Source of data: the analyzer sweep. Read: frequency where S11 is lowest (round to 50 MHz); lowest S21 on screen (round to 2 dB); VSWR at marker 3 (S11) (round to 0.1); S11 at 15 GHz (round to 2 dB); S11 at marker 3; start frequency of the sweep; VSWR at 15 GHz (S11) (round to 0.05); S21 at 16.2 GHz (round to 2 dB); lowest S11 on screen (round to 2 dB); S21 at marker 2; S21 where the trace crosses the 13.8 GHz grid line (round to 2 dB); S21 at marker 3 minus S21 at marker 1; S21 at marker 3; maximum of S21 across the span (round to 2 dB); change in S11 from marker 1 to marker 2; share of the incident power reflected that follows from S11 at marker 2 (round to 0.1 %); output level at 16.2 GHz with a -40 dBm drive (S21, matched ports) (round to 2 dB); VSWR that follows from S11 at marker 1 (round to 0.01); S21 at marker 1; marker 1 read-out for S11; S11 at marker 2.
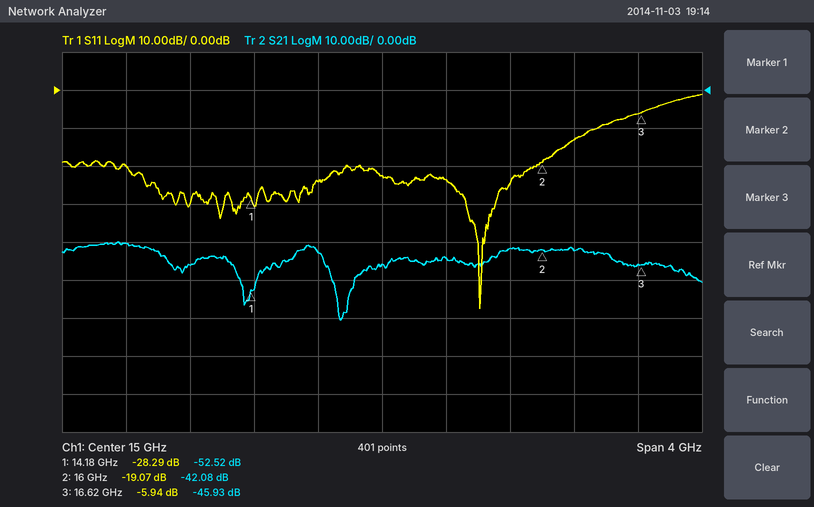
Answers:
15.60 GHz
-60 dB
3.0
-22 dB
-5.94 dB
13 GHz
1.15
-42 dB
-58 dB
-42.08 dB
-46 dB
6.59 dB
-45.93 dB
-40 dB
9.22 dB
1.2 %
-82 dBm
1.08
-52.52 dB
-28.29 dB
-19.07 dB
